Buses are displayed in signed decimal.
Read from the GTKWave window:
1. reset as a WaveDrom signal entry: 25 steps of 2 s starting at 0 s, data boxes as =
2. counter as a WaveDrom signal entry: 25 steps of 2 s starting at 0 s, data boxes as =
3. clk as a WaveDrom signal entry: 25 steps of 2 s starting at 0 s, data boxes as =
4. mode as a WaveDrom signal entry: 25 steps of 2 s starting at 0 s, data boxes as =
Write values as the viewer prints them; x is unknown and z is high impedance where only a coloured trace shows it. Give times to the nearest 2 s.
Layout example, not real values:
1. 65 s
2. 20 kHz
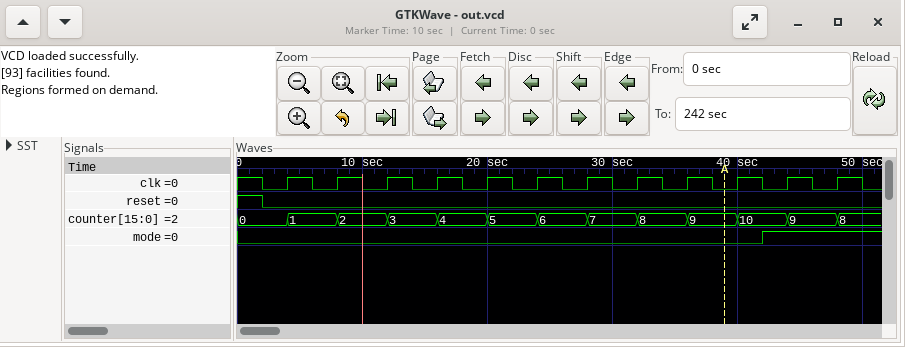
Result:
1. {name: 'reset', wave: '10.......................'}
2. {name: 'counter', wave: '=.=.=.=.=.=.=.=.=.=.=.=.=', data: '0 1 2 3 4 5 6 7 8 9 10 9 8'}
3. {name: 'clk', wave: '1010101010101010101010101'}
4. {name: 'mode', wave: '0....................1...'}
